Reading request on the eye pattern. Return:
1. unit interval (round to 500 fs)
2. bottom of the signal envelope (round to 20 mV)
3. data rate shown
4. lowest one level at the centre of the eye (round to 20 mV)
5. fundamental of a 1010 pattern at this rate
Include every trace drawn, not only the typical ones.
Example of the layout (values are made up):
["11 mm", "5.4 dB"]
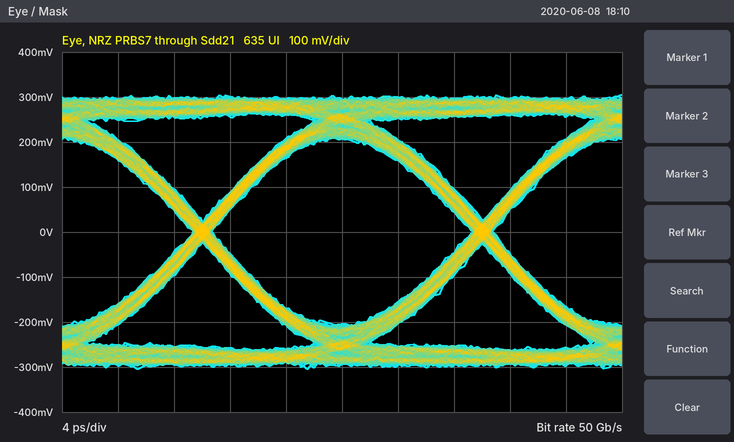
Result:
["20.0 ps", "-300 mV", "50 Gb/s", "200 mV", "25 GHz"]
